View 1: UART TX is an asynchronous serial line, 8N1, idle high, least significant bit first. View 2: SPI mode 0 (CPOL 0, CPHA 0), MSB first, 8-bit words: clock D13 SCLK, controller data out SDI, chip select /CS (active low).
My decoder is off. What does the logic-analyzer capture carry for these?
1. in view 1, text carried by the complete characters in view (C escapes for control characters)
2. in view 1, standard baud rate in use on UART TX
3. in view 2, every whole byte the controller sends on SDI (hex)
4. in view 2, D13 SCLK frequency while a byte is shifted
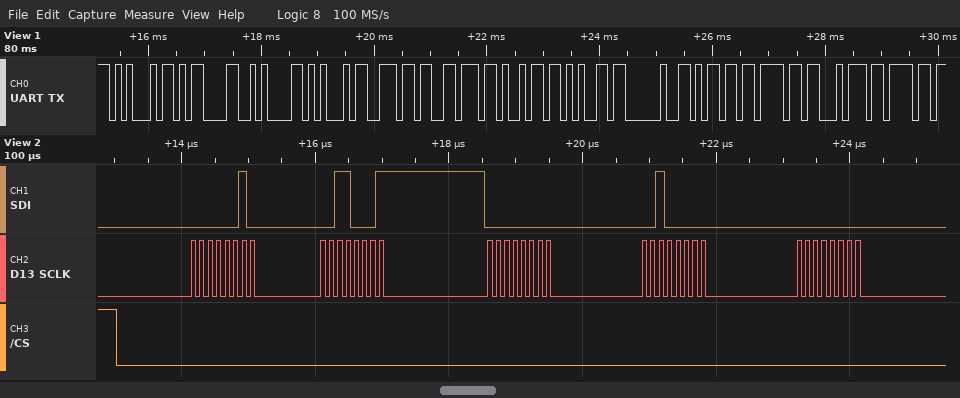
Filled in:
"E\r\nEnvie moto"
9600 baud
02 31 00 20 00
8 MHz
